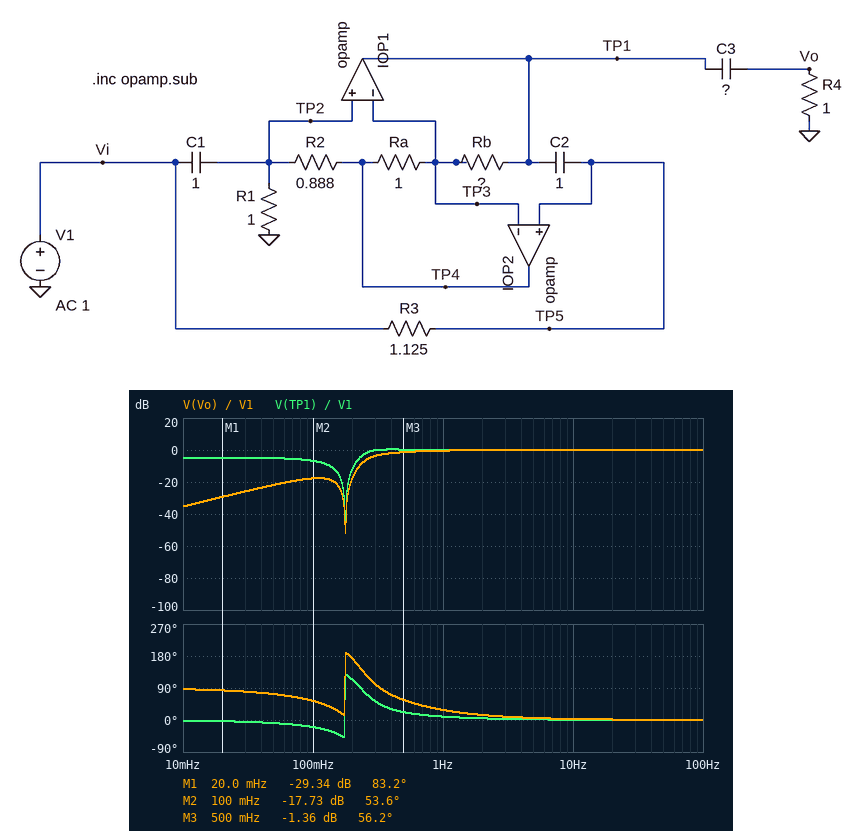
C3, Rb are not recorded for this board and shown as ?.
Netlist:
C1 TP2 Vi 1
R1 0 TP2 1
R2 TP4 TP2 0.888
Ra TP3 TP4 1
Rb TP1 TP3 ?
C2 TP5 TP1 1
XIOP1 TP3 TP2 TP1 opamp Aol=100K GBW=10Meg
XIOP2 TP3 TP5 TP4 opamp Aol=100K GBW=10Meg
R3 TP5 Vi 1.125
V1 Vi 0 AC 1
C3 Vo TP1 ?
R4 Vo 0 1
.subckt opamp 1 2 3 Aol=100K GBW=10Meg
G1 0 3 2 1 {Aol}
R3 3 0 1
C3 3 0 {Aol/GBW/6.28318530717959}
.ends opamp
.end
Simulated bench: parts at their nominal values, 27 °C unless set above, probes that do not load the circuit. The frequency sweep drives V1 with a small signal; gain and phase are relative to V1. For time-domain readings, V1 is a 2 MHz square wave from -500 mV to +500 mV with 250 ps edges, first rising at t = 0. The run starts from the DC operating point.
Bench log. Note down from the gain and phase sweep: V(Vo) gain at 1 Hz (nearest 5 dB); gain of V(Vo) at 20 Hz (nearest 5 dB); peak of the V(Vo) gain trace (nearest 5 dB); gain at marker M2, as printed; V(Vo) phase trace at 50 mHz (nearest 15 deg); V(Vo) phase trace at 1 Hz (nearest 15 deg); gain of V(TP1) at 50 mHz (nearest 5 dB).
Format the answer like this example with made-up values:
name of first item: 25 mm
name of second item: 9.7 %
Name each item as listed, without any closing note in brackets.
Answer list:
V(Vo) gain at 1 Hz: 0 dB
gain of V(Vo) at 20 Hz: 0 dB
peak of the V(Vo) gain trace: 0 dB
gain at marker M2, as printed: -17.73 dB
V(Vo) phase trace at 50 mHz: 75 deg
V(Vo) phase trace at 1 Hz: 30 deg
gain of V(TP1) at 50 mHz: -5 dB
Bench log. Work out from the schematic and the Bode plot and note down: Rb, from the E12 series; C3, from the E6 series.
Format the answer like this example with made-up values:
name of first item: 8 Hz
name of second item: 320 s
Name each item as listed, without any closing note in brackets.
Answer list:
Rb, from the E12 series: 0.47 Ω
C3, from the E6 series: 470 mF
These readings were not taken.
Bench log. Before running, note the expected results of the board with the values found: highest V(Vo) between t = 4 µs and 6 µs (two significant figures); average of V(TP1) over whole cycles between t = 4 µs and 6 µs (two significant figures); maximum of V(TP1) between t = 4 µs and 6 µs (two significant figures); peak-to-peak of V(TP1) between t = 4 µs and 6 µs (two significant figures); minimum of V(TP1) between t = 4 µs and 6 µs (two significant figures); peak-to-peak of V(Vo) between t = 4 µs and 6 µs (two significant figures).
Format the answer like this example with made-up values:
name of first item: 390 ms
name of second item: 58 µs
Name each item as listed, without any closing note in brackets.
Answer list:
highest V(Vo) between t = 4 µs and 6 µs: 1.2 V
average of V(TP1) over whole cycles between t = 4 µs and 6 µs: 210 mV
maximum of V(TP1) between t = 4 µs and 6 µs: 870 mV
peak-to-peak of V(TP1) between t = 4 µs and 6 µs: 1.3 V
minimum of V(TP1) between t = 4 µs and 6 µs: -450 mV
peak-to-peak of V(Vo) between t = 4 µs and 6 µs: 1.3 V
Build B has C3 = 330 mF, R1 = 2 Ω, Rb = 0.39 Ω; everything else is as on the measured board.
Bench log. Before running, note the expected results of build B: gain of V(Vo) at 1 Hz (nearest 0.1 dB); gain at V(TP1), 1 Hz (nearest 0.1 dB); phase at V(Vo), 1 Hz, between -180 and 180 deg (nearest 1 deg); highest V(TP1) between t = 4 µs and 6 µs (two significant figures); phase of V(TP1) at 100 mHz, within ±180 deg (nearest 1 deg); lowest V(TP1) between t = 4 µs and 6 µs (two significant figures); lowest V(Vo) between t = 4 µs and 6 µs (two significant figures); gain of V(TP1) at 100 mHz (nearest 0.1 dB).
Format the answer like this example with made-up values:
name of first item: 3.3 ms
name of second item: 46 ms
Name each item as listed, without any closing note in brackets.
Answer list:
gain of V(Vo) at 1 Hz: -0.8 dB
gain at V(TP1), 1 Hz: 0.1 dB
phase at V(Vo), 1 Hz, between -180 and 180 deg: 31 deg
highest V(TP1) between t = 4 µs and 6 µs: 730 mV
phase of V(TP1) at 100 mHz, within ±180 deg: -8 deg
lowest V(TP1) between t = 4 µs and 6 µs: -560 mV
lowest V(Vo) between t = 4 µs and 6 µs: -150 mV
gain of V(TP1) at 100 mHz: -2.1 dB
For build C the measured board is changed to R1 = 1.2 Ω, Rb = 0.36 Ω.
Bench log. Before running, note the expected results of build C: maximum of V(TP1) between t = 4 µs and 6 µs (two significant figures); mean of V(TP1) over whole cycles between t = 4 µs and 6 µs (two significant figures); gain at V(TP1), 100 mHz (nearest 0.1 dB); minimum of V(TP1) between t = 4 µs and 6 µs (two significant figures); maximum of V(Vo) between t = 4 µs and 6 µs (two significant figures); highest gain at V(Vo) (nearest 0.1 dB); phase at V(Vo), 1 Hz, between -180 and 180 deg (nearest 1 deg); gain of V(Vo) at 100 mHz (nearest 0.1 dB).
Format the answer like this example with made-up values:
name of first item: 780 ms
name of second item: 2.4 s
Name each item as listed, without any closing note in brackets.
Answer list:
maximum of V(TP1) between t = 4 µs and 6 µs: 770 mV
mean of V(TP1) over whole cycles between t = 4 µs and 6 µs: 130 mV
gain at V(TP1), 100 mHz: -3.4 dB
minimum of V(TP1) between t = 4 µs and 6 µs: -510 mV
maximum of V(Vo) between t = 4 µs and 6 µs: 1.1 V
highest gain at V(Vo): 0 dB
phase at V(Vo), 1 Hz, between -180 and 180 deg: 27 deg
gain of V(Vo) at 100 mHz: -14.4 dB
